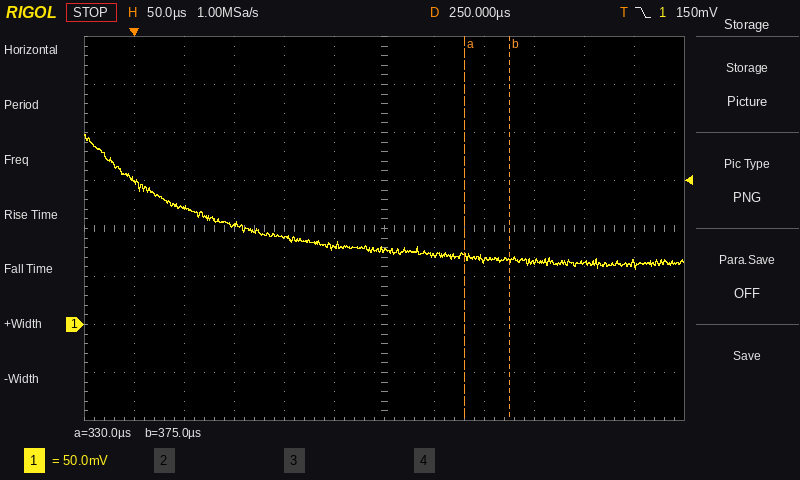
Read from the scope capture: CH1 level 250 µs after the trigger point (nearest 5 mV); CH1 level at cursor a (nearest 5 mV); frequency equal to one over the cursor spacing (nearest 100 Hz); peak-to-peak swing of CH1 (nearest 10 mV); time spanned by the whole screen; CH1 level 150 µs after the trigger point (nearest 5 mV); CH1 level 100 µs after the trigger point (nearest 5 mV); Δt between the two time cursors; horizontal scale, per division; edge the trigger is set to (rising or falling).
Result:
80 mV
70 mV
22.2 kHz
140 mV
600 µs
90 mV
105 mV
45 µs
50 µs
falling
